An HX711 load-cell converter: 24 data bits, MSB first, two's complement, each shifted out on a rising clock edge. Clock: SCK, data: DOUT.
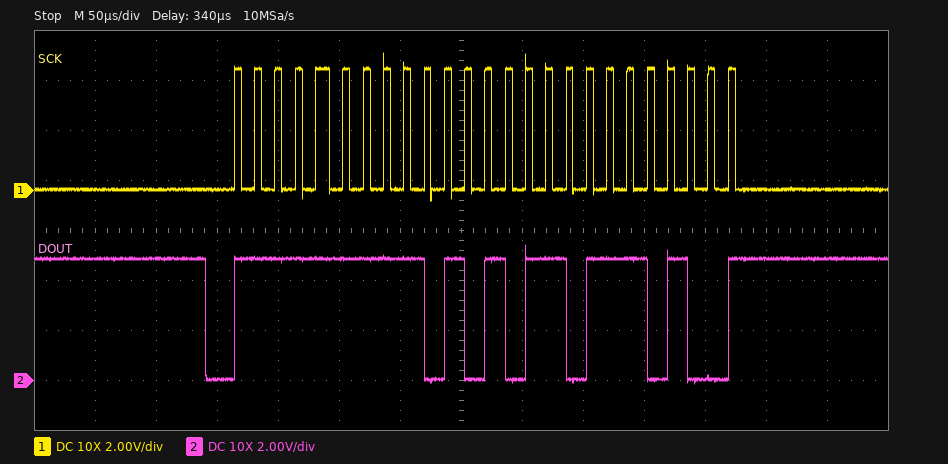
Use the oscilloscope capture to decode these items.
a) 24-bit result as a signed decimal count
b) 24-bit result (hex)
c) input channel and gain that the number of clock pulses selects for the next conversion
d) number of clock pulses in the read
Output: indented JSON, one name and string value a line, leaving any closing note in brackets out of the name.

{
  "24-bit result as a signed decimal count": "-21644",
  "24-bit result": "0xFFAB74",
  "input channel and gain that the number of clock pulses selects for the next conversion": "channel A, gain 128",
  "number of clock pulses in the read": "25"
}
